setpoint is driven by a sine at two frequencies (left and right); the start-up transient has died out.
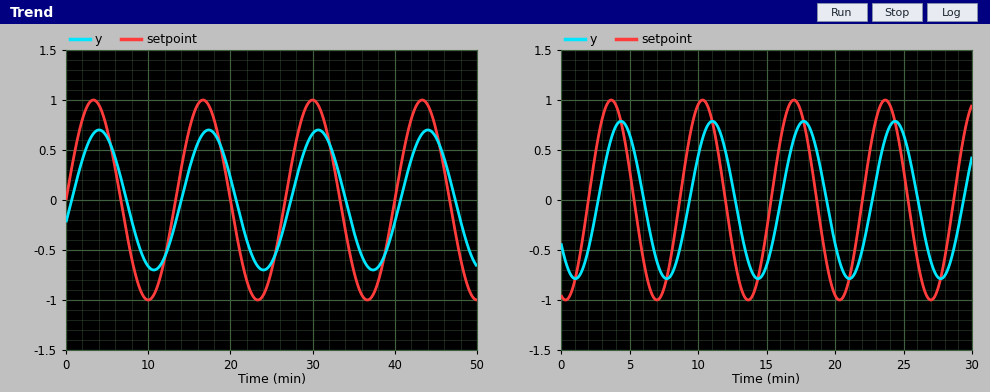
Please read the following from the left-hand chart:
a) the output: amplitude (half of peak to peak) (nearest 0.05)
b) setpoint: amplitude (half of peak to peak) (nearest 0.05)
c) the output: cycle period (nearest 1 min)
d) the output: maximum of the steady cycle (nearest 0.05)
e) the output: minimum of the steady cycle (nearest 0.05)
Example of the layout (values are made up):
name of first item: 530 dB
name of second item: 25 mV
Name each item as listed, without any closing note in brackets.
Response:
the output: amplitude (half of peak to peak): 0.70
setpoint: amplitude (half of peak to peak): 1.00
the output: cycle period: 13 min
the output: maximum of the steady cycle: 0.70
the output: minimum of the steady cycle: -0.70
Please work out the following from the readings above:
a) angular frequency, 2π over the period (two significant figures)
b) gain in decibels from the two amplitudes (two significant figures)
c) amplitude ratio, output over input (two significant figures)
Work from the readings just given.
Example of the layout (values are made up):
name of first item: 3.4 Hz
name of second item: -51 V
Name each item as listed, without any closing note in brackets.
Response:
angular frequency, 2π over the period: 0.48 rad/min
gain in decibels from the two amplitudes: -3.1 dB
amplitude ratio, output over input: 0.70
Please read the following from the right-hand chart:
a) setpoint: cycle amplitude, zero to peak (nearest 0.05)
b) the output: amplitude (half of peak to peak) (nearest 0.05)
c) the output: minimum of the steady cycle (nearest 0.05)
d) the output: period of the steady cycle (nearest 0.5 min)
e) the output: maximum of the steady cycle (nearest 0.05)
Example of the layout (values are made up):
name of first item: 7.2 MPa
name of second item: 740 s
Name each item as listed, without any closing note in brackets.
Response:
setpoint: cycle amplitude, zero to peak: 1.00
the output: amplitude (half of peak to peak): 0.80
the output: minimum of the steady cycle: -0.80
the output: period of the steady cycle: 6.5 min
the output: maximum of the steady cycle: 0.80
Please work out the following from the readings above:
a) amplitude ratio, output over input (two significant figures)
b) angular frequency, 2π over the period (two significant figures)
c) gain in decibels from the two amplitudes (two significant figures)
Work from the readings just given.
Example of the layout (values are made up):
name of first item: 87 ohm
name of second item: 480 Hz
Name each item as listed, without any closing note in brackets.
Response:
amplitude ratio, output over input: 0.80
angular frequency, 2π over the period: 0.97 rad/min
gain in decibels from the two amplitudes: -1.9 dB
